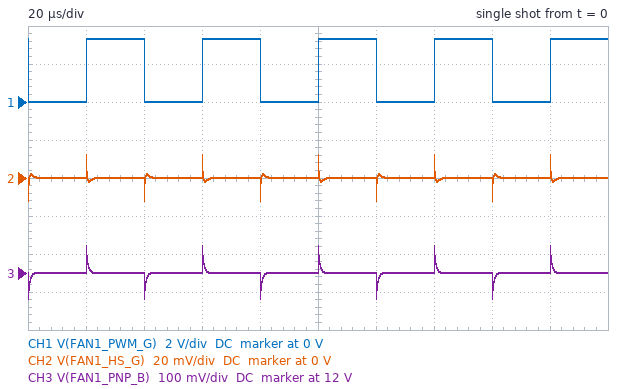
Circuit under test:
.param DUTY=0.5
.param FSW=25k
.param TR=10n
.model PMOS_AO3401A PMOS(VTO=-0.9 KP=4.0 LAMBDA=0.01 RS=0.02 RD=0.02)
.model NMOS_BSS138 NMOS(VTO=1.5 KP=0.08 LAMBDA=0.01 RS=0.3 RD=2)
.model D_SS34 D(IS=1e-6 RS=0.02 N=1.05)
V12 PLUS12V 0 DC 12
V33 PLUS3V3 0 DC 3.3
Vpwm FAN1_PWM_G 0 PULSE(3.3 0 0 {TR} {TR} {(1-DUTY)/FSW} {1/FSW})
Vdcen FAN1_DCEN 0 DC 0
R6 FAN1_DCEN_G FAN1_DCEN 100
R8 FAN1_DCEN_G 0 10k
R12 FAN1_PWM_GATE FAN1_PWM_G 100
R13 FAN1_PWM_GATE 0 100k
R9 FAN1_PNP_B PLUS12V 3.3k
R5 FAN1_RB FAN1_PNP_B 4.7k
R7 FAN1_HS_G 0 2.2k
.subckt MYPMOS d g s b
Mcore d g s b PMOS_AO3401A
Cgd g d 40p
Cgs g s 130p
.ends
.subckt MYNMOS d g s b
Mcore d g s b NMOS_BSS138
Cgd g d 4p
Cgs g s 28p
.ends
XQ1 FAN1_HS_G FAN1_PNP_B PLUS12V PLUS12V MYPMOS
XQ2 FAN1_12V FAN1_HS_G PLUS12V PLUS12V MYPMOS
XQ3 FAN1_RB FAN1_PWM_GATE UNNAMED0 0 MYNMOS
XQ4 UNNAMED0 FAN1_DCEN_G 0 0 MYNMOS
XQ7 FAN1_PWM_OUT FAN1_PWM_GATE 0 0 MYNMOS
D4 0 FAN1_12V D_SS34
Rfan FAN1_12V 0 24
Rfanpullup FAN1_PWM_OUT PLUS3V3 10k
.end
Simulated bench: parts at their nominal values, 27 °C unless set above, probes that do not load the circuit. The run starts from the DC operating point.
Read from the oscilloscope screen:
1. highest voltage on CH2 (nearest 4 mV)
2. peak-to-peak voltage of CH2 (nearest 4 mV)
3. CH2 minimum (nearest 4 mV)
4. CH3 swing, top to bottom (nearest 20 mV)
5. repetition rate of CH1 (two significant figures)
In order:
12 mV
24 mV
-12 mV
140 mV
25 kHz
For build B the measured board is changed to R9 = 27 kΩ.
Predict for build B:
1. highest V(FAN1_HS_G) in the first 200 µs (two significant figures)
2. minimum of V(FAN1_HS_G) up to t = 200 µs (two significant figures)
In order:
13 mV
-13 mV
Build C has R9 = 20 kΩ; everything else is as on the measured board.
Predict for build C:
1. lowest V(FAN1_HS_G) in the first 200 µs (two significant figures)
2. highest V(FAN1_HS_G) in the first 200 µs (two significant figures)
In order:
-13 mV
13 mV
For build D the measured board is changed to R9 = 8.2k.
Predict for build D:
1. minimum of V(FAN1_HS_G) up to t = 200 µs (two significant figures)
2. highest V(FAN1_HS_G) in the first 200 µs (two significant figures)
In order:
-13 mV
13 mV
